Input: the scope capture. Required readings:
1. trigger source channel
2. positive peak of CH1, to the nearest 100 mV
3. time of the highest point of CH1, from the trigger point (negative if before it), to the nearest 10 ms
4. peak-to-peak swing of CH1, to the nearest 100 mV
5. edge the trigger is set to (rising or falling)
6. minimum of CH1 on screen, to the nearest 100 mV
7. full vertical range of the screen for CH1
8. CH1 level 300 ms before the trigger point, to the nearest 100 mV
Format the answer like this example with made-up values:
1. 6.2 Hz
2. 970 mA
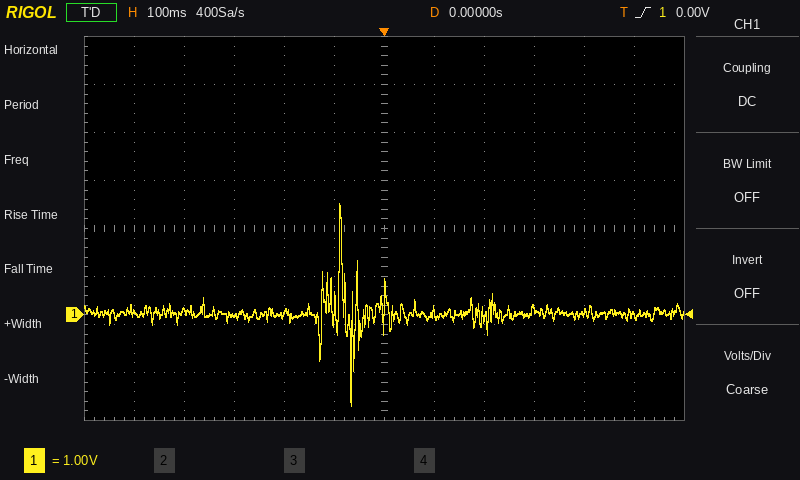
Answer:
1. CH1
2. 2.3 V
3. -90 ms
4. 4.2 V
5. rising
6. -1.9 V
7. 8 V
8. 0.0 V
